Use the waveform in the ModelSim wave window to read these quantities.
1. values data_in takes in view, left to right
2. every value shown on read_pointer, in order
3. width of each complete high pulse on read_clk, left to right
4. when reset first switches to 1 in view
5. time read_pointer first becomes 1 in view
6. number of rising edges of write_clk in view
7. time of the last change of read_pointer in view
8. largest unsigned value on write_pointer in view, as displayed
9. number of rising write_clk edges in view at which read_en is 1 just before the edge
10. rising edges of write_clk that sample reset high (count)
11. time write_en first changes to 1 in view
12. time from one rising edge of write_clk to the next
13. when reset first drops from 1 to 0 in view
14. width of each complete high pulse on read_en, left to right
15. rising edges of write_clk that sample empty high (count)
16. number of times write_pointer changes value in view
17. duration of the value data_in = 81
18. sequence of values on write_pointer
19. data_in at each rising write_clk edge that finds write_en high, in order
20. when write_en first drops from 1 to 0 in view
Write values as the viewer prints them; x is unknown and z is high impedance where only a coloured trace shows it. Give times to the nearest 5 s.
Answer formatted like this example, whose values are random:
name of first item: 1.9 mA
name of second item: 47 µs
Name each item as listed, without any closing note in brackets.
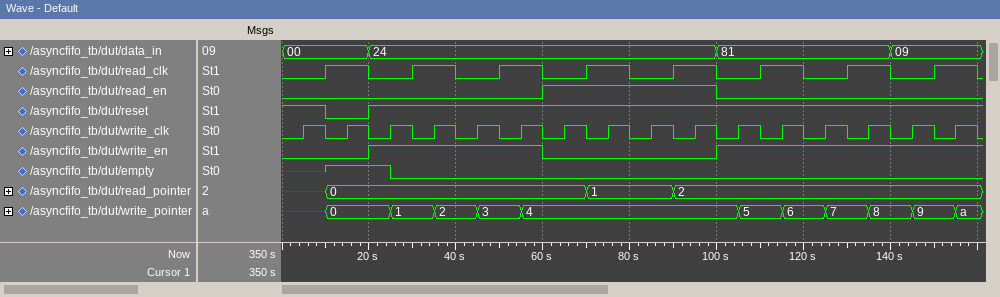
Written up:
values data_in takes in view, left to right: 00, 24, 81, 09
every value shown on read_pointer, in order: x, 0, 1, 2
width of each complete high pulse on read_clk, left to right: 10 s, 10 s, 10 s, 10 s, 10 s, 10 s, 10 s, 10 s
when reset first switches to 1 in view: 20 s
time read_pointer first becomes 1 in view: 70 s
number of rising edges of write_clk in view: 16
time of the last change of read_pointer in view: 90 s
largest unsigned value on write_pointer in view, as displayed: a
number of rising write_clk edges in view at which read_en is 1 just before the edge: 4
rising edges of write_clk that sample reset high: 15
time write_en first changes to 1 in view: 20 s
time from one rising edge of write_clk to the next: 10 s
when reset first drops from 1 to 0 in view: 10 s
width of each complete high pulse on read_en, left to right: 40 s
rising edges of write_clk that sample empty high: 2
number of times write_pointer changes value in view: 11
duration of the value data_in = 81: 40 s
sequence of values on write_pointer: x, 0, 1, 2, 3, 4, 5, 6, 7, 8, 9, a
data_in at each rising write_clk edge that finds write_en high, in order: 24, 24, 24, 24, 81, 81, 81, 81, 09, 09
when write_en first drops from 1 to 0 in view: 60 s
